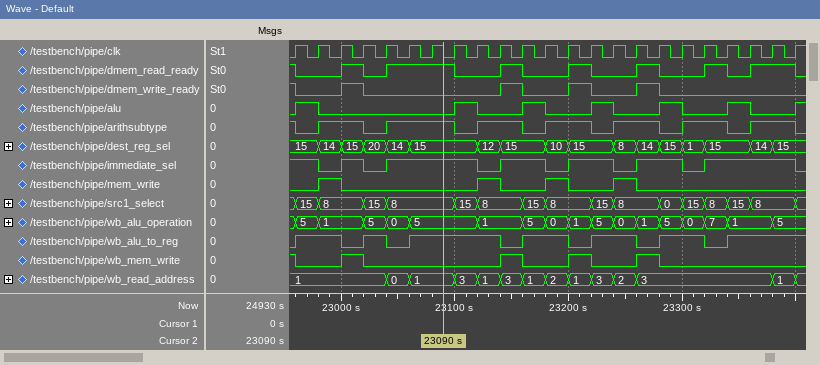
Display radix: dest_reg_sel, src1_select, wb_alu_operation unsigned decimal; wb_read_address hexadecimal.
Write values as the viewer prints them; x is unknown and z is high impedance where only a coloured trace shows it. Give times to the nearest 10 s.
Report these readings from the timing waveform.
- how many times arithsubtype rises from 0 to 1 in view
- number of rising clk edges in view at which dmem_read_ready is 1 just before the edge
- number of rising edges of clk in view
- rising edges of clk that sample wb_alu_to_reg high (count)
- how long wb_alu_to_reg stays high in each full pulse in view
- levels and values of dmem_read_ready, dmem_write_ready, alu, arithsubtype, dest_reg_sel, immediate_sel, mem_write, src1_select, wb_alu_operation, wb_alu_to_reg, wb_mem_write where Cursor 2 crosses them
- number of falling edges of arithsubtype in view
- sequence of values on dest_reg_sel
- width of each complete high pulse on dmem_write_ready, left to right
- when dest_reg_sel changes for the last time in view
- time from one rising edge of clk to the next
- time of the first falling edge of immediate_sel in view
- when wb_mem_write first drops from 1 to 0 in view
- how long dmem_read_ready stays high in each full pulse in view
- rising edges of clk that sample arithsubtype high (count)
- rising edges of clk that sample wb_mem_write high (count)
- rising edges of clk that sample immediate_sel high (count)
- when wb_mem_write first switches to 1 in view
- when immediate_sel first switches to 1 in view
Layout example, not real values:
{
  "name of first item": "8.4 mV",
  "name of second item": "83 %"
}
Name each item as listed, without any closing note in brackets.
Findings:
{
  "how many times arithsubtype rises from 0 to 1 in view": "7",
  "number of rising clk edges in view at which dmem_read_ready is 1 just before the edge": "11",
  "number of rising edges of clk in view": "23",
  "rising edges of clk that sample wb_alu_to_reg high": "16",
  "how long wb_alu_to_reg stays high in each full pulse in view": "40 s, 20 s, 80 s, 40 s, 40 s, 40 s",
  "levels and values of dmem_read_ready, dmem_write_ready, alu, arithsubtype, dest_reg_sel, immediate_sel, mem_write, src1_select, wb_alu_operation, wb_alu_to_reg, wb_mem_write where Cursor 2 crosses them": "dmem_read_ready=1, dmem_write_ready=0, alu=0, arithsubtype=1, dest_reg_sel=15, immediate_sel=1, mem_write=0, src1_select=8, wb_alu_operation=5, wb_alu_to_reg=1, wb_mem_write=0",
  "number of falling edges of arithsubtype in view": "8",
  "sequence of values on dest_reg_sel": "15, 14, 15, 20, 14, 15, 12, 15, 10, 15, 8, 14, 15, 1, 15, 14, 15",
  "width of each complete high pulse on dmem_write_ready, left to right": "20 s, 20 s, 20 s, 20 s",
  "when dest_reg_sel changes for the last time in view": "23380 s",
  "time from one rising edge of clk to the next": "20 s",
  "time of the first falling edge of immediate_sel in view": "22980 s",
  "when wb_mem_write first drops from 1 to 0 in view": "22960 s",
  "how long dmem_read_ready stays high in each full pulse in view": "20 s, 60 s, 20 s, 20 s, 20 s, 20 s, 40 s",
  "rising edges of clk that sample arithsubtype high": "16",
  "rising edges of clk that sample wb_mem_write high": "5",
  "rising edges of clk that sample immediate_sel high": "17",
  "when wb_mem_write first switches to 1 in view": "23000 s",
  "when immediate_sel first switches to 1 in view": "23000 s"
}
